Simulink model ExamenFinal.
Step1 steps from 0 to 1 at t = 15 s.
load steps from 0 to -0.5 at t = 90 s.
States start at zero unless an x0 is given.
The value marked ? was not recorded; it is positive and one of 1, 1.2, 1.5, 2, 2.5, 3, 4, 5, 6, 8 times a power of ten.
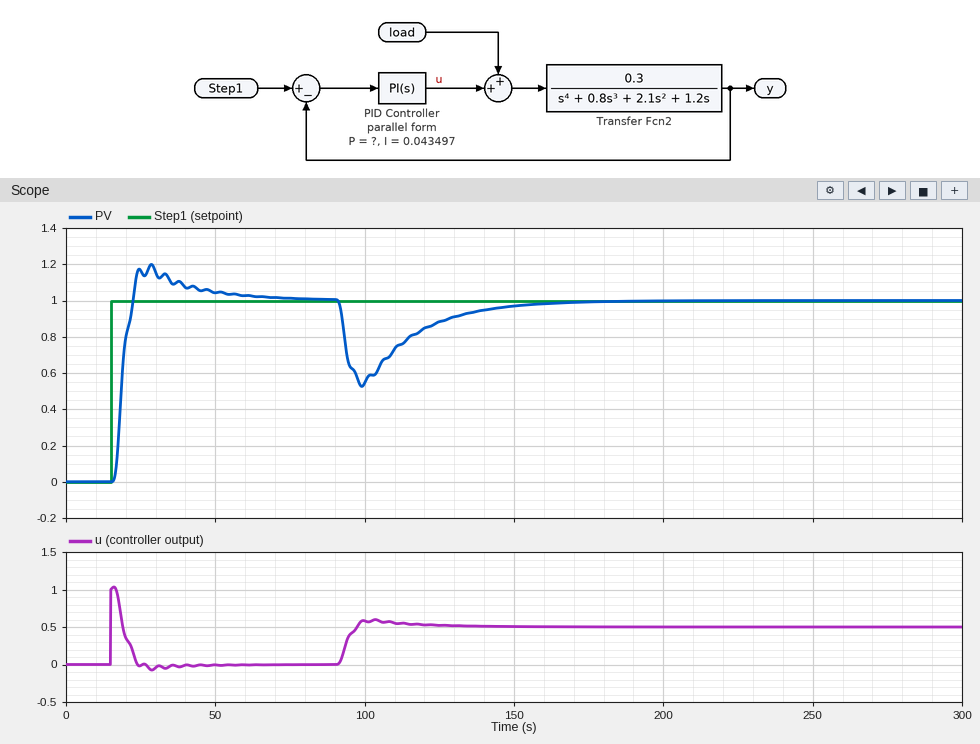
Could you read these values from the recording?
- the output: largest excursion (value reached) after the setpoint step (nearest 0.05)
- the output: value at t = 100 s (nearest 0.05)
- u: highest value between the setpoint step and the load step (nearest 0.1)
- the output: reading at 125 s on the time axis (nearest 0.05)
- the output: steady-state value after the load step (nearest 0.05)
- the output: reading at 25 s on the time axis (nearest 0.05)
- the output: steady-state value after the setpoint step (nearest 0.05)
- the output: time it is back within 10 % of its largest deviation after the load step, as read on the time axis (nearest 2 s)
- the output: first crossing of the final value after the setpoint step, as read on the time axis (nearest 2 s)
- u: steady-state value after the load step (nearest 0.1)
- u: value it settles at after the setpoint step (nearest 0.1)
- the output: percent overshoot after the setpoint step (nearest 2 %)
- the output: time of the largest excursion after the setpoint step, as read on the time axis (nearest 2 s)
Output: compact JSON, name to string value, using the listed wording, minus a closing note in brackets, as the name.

{"the output: largest excursion (value reached) after the setpoint step": "1.20", "the output: value at t = 100 s": "0.55", "u: highest value between the setpoint step and the load step": "1.0", "the output: reading at 125 s on the time axis": "0.90", "the output: steady-state value after the load step": "1.00", "the output: reading at 25 s on the time axis": "1.15", "the output: steady-state value after the setpoint step": "1.00", "the output: time it is back within 10 % of its largest deviation after the load step, as read on the time axis": "142 s", "the output: first crossing of the final value after the setpoint step, as read on the time axis": "22 s", "u: steady-state value after the load step": "0.5", "u: value it settles at after the setpoint step": "0.0", "the output: percent overshoot after the setpoint step": "20 %", "the output: time of the largest excursion after the setpoint step, as read on the time axis": "28 s"}
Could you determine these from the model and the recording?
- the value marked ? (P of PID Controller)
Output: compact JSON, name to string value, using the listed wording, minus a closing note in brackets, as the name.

{"the value marked ?": "1"}
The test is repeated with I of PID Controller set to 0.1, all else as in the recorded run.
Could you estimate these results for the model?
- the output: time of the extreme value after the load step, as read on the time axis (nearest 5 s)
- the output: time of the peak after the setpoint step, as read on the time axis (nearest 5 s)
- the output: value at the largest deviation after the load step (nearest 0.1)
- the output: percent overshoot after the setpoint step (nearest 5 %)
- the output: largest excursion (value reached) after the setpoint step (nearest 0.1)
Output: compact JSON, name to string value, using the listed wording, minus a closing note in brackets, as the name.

{"the output: time of the extreme value after the load step, as read on the time axis": "100 s", "the output: time of the peak after the setpoint step, as read on the time axis": "25 s", "the output: value at the largest deviation after the load step": "0.6", "the output: percent overshoot after the setpoint step": "35 %", "the output: largest excursion (value reached) after the setpoint step": "1.3"}
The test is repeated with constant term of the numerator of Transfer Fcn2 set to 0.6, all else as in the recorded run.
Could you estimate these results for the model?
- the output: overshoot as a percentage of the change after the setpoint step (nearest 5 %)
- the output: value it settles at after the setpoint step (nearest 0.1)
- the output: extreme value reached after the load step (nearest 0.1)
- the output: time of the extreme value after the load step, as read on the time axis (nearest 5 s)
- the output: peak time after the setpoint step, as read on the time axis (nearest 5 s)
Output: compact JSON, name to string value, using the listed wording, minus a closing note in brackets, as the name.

{"the output: overshoot as a percentage of the change after the setpoint step": "35 %", "the output: value it settles at after the setpoint step": "1.0", "the output: extreme value reached after the load step": "0.4", "the output: time of the extreme value after the load step, as read on the time axis": "95 s", "the output: peak time after the setpoint step, as read on the time axis": "20 s"}
